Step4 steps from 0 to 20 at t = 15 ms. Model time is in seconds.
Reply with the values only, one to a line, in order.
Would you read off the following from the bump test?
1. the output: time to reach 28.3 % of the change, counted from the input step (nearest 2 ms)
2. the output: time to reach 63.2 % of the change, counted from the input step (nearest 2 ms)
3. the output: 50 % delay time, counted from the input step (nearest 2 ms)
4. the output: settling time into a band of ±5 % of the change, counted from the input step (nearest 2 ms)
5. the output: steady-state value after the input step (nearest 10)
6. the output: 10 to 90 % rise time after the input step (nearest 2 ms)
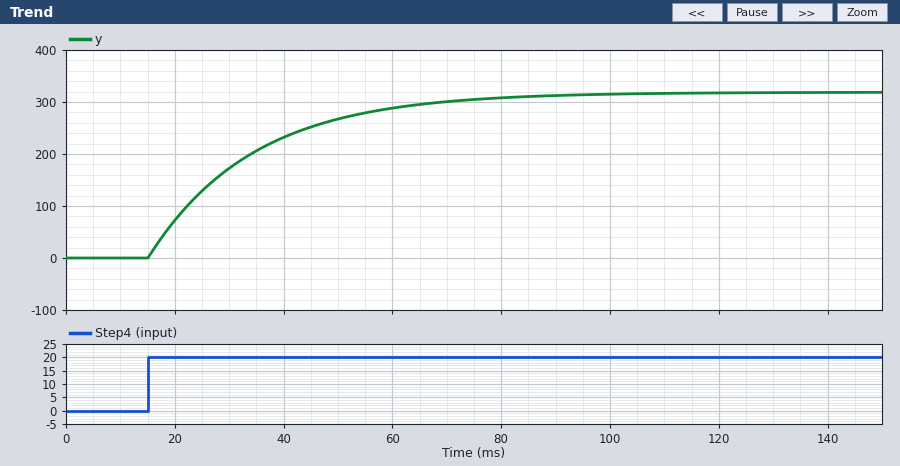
6 ms
20 ms
14 ms
58 ms
320
42 ms
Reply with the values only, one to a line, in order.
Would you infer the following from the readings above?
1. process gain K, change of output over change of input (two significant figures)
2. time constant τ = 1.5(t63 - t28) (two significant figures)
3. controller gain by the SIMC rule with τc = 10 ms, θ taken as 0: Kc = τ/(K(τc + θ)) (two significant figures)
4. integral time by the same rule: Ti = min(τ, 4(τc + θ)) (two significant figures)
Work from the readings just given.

16
21 ms
0.13
21 ms
